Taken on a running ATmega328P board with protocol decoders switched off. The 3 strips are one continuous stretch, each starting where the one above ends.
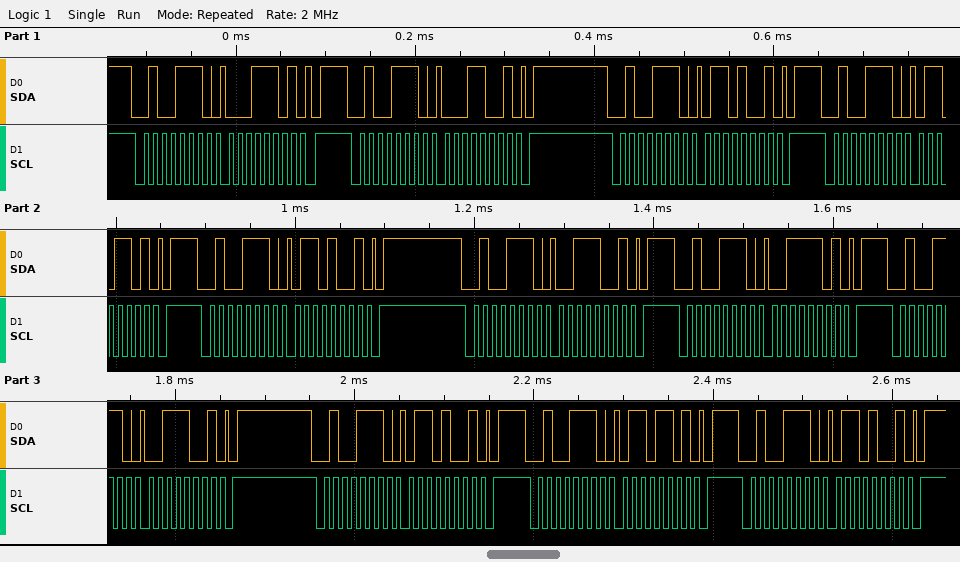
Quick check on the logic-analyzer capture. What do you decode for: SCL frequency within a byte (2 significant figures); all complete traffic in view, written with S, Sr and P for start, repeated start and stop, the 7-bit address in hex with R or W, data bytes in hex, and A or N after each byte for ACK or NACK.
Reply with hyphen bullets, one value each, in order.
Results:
- 100 kHz
- S 27W A 1D A P S 27W A 19 A P S 27W A 69 A P S 27W A 6D A P S 27W A 69 A P S 27W A 39 A P S 27W A 3D A P S 27W A 39 A P S 27W A 69 A P S 27W A 6D A P S 27W A 69 A P
